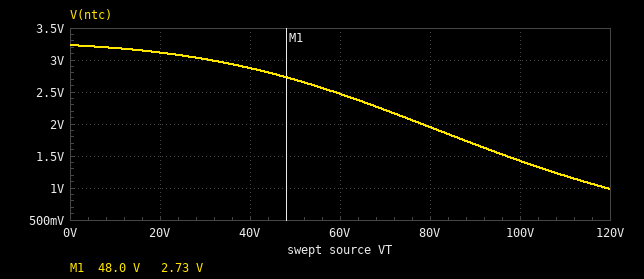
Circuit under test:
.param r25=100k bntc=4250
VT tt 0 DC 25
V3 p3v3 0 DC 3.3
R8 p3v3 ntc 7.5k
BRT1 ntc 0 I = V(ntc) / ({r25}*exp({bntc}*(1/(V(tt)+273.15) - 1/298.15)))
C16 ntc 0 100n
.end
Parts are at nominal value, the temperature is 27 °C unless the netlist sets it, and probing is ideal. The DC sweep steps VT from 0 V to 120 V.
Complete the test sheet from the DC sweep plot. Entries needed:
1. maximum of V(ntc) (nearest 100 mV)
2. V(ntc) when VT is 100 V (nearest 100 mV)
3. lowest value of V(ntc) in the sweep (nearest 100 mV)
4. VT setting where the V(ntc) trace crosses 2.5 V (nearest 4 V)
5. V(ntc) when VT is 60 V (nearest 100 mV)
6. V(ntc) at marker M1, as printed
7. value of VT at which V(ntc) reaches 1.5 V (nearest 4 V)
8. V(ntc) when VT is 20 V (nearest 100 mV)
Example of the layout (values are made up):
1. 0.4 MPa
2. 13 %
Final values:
1. 3.2 V
2. 1.4 V
3. 1.0 V
4. 60 V
5. 2.5 V
6. 2.73 V
7. 96 V
8. 3.1 V
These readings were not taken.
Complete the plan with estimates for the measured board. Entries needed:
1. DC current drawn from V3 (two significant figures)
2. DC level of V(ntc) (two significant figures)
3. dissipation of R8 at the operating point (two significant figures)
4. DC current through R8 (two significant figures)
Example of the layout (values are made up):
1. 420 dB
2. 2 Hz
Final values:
1. 31 µA
2. 3.1 V
3. 7.1 µW
4. 31 µA
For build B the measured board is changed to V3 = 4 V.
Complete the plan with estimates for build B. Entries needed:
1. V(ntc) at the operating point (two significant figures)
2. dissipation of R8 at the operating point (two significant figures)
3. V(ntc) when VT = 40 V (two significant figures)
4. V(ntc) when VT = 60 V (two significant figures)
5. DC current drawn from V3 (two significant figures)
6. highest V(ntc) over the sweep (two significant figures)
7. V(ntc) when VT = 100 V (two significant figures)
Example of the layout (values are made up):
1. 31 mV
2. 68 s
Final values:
1. 3.7 V
2. 10 µW
3. 3.5 V
4. 3.0 V
5. 37 µA
6. 3.9 V
7. 1.7 V
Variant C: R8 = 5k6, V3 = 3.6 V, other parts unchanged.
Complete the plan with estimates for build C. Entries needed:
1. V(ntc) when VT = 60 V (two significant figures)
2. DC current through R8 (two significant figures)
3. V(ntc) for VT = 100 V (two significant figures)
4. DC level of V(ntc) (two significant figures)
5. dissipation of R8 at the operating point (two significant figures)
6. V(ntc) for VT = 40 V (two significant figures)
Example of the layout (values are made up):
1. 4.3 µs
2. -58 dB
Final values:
1. 2.9 V
2. 34 µA
3. 1.8 V
4. 3.4 V
5. 6.5 µW
6. 3.2 V
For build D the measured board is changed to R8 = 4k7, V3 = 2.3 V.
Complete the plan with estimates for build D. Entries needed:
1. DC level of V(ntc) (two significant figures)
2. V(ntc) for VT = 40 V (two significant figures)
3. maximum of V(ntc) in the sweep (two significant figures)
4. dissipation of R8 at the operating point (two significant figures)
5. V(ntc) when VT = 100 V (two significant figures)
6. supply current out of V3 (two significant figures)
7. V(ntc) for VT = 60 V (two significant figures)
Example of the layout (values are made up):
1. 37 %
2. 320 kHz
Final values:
1. 2.2 V
2. 2.1 V
3. 2.3 V
4. 2.3 µW
5. 1.3 V
6. 22 µA
7. 1.9 V
